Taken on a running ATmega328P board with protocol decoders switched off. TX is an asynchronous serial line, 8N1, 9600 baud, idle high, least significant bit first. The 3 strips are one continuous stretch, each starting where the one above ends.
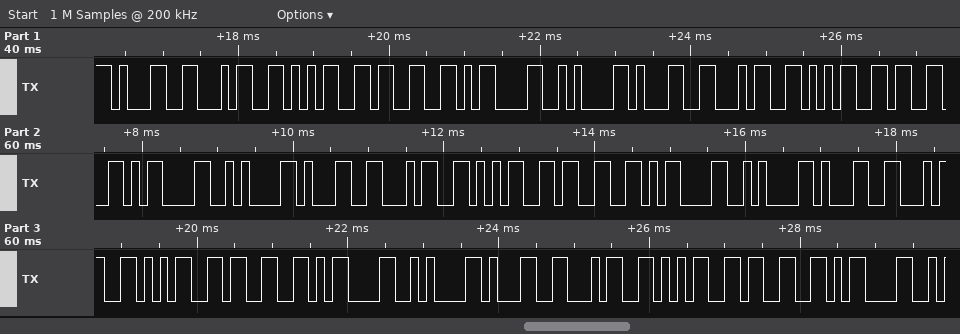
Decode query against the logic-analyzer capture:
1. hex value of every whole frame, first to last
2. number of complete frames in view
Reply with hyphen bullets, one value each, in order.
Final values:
- 0x31 0x34 0x35 0x33 0x0D 0x0A 0x31 0x34 0x35 0x33 0x0D 0x0A 0x31 0x34 0x35 0x33 0x0D 0x0A 0x31 0x34 0x35 0x33 0x0D 0x0A 0x31 0x34 0x35 0x33 0x0D
- 29
